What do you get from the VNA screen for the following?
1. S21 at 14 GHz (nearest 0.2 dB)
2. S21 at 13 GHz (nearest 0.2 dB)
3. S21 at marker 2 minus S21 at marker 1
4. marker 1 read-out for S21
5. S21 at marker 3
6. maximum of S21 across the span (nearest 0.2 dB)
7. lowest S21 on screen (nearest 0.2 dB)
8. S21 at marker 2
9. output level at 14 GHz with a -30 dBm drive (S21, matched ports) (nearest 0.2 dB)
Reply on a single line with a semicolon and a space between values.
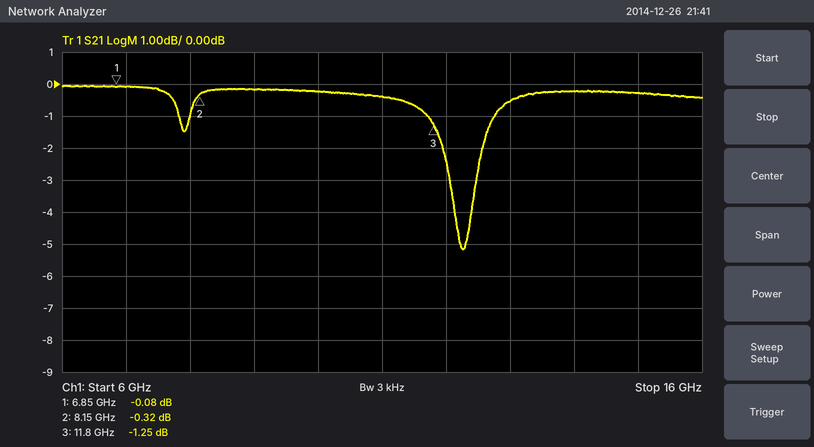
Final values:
-0.2 dB; -0.6 dB; -0.24 dB; -0.08 dB; -1.25 dB; 0.0 dB; -5.2 dB; -0.32 dB; -30.2 dBm
